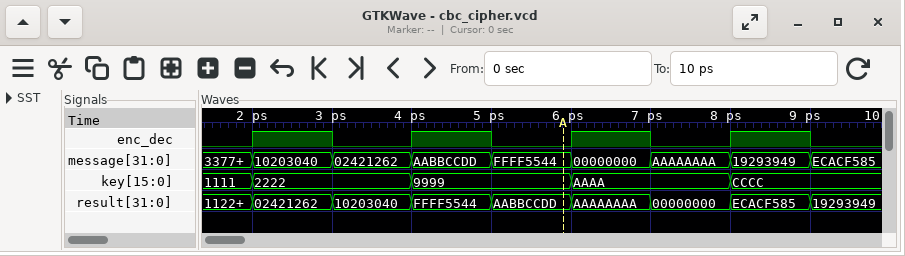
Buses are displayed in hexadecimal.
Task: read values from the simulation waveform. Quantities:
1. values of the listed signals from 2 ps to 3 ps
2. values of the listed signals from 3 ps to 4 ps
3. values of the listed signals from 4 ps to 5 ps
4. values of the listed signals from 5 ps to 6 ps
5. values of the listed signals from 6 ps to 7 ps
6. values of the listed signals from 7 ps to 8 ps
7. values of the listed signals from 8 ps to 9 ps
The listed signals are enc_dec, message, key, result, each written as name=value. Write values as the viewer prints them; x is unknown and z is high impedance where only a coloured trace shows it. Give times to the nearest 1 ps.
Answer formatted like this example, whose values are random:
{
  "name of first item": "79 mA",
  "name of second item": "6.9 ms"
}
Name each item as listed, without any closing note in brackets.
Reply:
{
  "values of the listed signals from 2 ps to 3 ps": "enc_dec=1, message=10203040, key=2222, result=02421262",
  "values of the listed signals from 3 ps to 4 ps": "enc_dec=0, message=02421262, key=2222, result=10203040",
  "values of the listed signals from 4 ps to 5 ps": "enc_dec=1, message=AABBCCDD, key=9999, result=FFFF5544",
  "values of the listed signals from 5 ps to 6 ps": "enc_dec=0, message=FFFF5544, key=9999, result=AABBCCDD",
  "values of the listed signals from 6 ps to 7 ps": "enc_dec=1, message=00000000, key=AAAA, result=AAAAAAAA",
  "values of the listed signals from 7 ps to 8 ps": "enc_dec=0, message=AAAAAAAA, key=AAAA, result=00000000",
  "values of the listed signals from 8 ps to 9 ps": "enc_dec=1, message=19293949, key=CCCC, result=ECACF585"
}
